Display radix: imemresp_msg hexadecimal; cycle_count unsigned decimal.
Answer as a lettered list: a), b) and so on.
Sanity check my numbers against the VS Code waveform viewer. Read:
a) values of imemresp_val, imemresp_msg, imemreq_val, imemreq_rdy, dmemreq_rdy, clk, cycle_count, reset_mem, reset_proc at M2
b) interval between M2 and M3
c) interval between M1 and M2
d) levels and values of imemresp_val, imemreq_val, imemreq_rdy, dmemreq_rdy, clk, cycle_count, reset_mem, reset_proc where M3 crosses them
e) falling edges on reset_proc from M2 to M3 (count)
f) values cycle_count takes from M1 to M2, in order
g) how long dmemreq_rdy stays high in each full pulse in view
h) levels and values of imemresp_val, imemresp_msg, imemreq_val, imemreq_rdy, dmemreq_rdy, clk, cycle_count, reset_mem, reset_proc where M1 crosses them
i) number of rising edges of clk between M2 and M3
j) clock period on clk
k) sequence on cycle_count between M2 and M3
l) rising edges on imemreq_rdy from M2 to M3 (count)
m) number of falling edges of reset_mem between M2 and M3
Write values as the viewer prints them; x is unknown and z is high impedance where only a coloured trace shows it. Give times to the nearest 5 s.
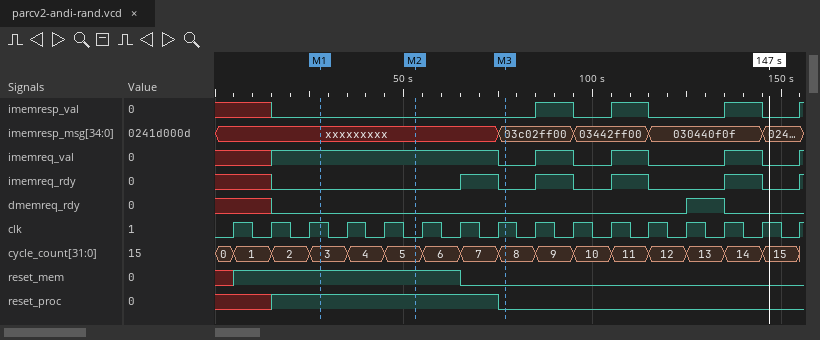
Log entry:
a) imemresp_val=0, imemresp_msg=xxxxxxxxx, imemreq_val=1, imemreq_rdy=0, dmemreq_rdy=0, clk=0, cycle_count=5, reset_mem=1, reset_proc=1
b) 25 s
c) 25 s
d) imemresp_val=0, imemreq_val=0, imemreq_rdy=0, dmemreq_rdy=0, clk=1, cycle_count=8, reset_mem=0, reset_proc=0
e) 1
f) 3, 4, 5
g) 10 s
h) imemresp_val=0, imemresp_msg=xxxxxxxxx, imemreq_val=1, imemreq_rdy=0, dmemreq_rdy=0, clk=1, cycle_count=3, reset_mem=1, reset_proc=1
i) 3
j) 10 s
k) 5, 6, 7, 8
l) 1
m) 1
